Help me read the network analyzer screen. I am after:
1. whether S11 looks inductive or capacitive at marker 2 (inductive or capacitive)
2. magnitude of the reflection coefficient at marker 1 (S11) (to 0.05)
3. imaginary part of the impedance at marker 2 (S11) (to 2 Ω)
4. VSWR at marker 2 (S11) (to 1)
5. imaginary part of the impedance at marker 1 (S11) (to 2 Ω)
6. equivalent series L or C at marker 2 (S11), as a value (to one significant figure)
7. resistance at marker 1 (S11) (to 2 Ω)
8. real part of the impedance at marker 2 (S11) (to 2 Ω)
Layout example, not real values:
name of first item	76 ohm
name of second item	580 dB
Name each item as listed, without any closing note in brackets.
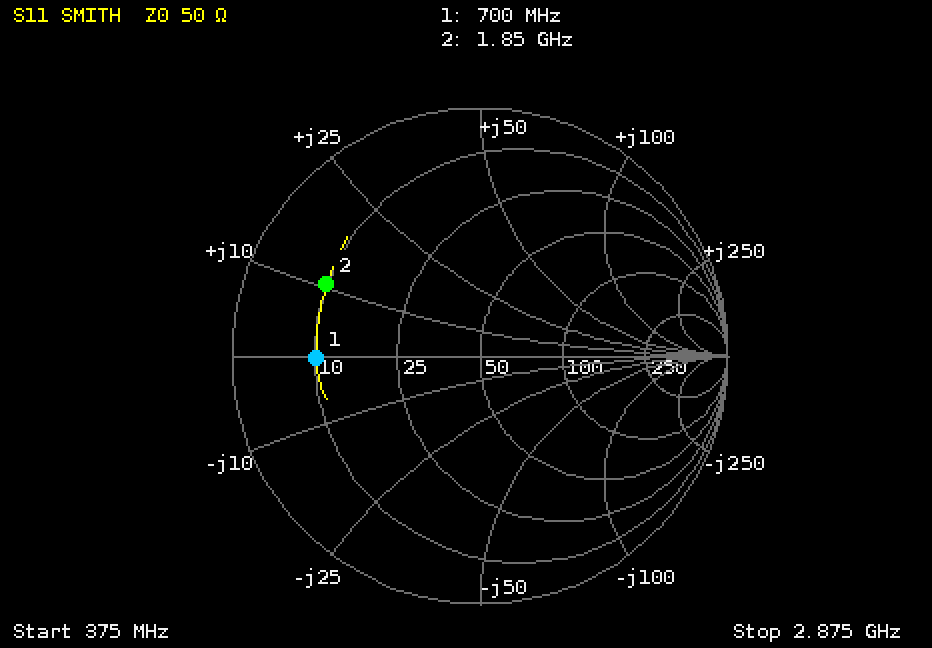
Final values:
whether S11 looks inductive or capacitive at marker 2	inductive
magnitude of the reflection coefficient at marker 1 (S11)	0.65
imaginary part of the impedance at marker 2 (S11)	+10 Ω
VSWR at marker 2 (S11)	5
imaginary part of the impedance at marker 1 (S11)	0 Ω
equivalent series L or C at marker 2 (S11), as a value	900 pH
resistance at marker 1 (S11)	10 Ω
real part of the impedance at marker 2 (S11)	10 Ω
